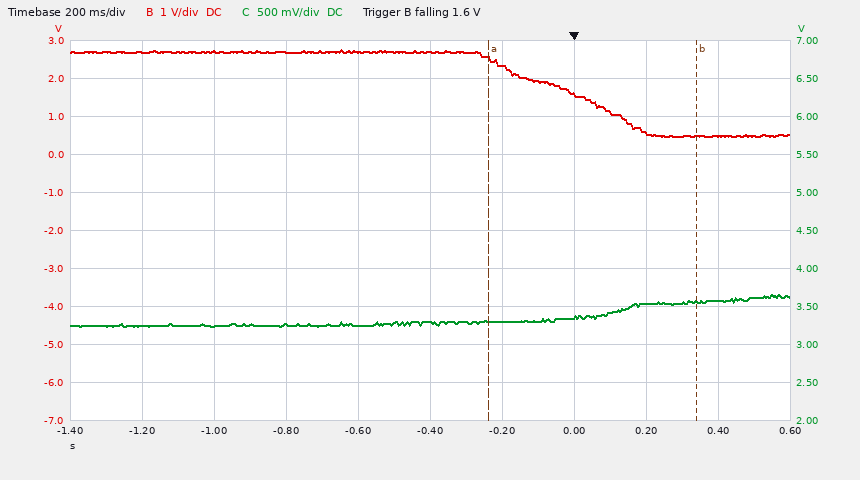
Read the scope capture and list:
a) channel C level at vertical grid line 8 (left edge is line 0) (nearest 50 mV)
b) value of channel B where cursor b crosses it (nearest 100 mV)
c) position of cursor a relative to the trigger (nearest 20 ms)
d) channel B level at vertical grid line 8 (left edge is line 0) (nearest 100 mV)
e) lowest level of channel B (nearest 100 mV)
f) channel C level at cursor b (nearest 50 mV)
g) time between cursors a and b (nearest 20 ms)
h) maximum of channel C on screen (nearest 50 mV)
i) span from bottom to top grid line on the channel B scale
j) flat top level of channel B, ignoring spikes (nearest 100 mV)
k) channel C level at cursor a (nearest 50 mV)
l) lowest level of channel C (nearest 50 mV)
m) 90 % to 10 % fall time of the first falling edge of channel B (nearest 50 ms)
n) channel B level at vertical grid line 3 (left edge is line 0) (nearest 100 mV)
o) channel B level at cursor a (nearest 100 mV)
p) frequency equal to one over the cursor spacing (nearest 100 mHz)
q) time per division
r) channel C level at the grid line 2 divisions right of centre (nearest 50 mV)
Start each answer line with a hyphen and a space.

- 3.55 V
- 500 mV
- -240 ms
- 600 mV
- 500 mV
- 3.55 V
- 580 ms
- 3.65 V
- 10 V
- 2.7 V
- 3.30 V
- 3.25 V
- 400 ms
- 2.7 V
- 2.5 V
- 1.7 Hz
- 200 ms
- 3.35 V
